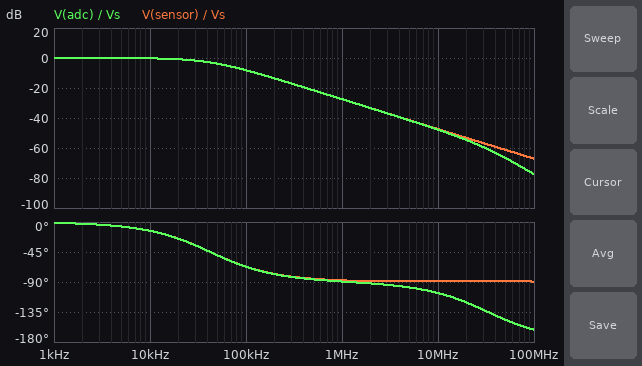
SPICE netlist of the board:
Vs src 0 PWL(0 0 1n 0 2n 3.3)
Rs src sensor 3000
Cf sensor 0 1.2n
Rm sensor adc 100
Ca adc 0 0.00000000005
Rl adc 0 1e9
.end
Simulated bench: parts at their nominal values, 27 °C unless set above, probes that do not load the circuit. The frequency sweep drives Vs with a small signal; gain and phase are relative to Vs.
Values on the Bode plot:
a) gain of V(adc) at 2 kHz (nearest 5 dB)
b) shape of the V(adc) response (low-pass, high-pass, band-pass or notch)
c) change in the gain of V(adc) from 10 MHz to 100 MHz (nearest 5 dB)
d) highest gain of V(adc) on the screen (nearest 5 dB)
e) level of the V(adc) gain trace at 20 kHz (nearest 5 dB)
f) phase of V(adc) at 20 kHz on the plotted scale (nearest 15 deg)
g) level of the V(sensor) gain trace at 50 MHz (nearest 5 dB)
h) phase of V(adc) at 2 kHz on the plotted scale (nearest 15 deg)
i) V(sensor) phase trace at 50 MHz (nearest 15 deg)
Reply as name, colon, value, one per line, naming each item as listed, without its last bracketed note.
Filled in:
gain of V(adc) at 2 kHz: 0 dB
shape of the V(adc) response: low-pass
change in the gain of V(adc) from 10 MHz to 100 MHz: -30 dB
highest gain of V(adc) on the screen: 0 dB
level of the V(adc) gain trace at 20 kHz: 0 dB
phase of V(adc) at 20 kHz on the plotted scale: -30 deg
level of the V(sensor) gain trace at 50 MHz: -60 dB
phase of V(adc) at 2 kHz on the plotted scale: 0 deg
V(sensor) phase trace at 50 MHz: -90 deg
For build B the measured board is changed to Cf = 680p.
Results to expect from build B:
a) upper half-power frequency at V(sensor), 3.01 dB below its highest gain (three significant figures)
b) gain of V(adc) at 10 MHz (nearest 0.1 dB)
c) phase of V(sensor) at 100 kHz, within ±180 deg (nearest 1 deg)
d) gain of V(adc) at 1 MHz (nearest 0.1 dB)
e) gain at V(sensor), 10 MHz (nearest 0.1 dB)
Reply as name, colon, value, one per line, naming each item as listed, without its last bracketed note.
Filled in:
upper half-power frequency at V(sensor), 3.01 dB below its highest gain: 72.7 kHz
gain of V(adc) at 10 MHz: -43.1 dB
phase of V(sensor) at 100 kHz, within ±180 deg: -54 deg
gain of V(adc) at 1 MHz: -22.8 dB
gain at V(sensor), 10 MHz: -42.7 dB
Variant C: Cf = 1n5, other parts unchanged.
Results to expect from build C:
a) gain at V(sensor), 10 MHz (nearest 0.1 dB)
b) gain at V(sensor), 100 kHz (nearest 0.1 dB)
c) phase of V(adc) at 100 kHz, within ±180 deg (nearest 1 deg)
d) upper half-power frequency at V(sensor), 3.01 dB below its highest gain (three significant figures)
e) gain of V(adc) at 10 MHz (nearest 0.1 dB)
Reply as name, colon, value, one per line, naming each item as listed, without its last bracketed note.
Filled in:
gain at V(sensor), 10 MHz: -49.3 dB
gain at V(sensor), 100 kHz: -9.8 dB
phase of V(adc) at 100 kHz, within ±180 deg: -71 deg
upper half-power frequency at V(sensor), 3.01 dB below its highest gain: 34.2 kHz
gain of V(adc) at 10 MHz: -49.7 dB
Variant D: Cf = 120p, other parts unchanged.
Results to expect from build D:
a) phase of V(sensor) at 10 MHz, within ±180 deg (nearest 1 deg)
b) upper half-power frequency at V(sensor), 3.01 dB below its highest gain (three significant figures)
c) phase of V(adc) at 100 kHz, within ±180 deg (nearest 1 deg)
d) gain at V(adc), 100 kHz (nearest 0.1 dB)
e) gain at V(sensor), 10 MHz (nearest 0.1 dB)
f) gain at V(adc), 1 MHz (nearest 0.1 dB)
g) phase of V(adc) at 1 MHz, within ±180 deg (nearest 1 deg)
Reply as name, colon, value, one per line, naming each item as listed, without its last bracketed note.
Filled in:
phase of V(sensor) at 10 MHz, within ±180 deg: -83 deg
upper half-power frequency at V(sensor), 3.01 dB below its highest gain: 311 kHz
phase of V(adc) at 100 kHz, within ±180 deg: -18 deg
gain at V(adc), 100 kHz: -0.4 dB
gain at V(sensor), 10 MHz: -29.9 dB
gain at V(adc), 1 MHz: -10.5 dB
phase of V(adc) at 1 MHz, within ±180 deg: -74 deg
